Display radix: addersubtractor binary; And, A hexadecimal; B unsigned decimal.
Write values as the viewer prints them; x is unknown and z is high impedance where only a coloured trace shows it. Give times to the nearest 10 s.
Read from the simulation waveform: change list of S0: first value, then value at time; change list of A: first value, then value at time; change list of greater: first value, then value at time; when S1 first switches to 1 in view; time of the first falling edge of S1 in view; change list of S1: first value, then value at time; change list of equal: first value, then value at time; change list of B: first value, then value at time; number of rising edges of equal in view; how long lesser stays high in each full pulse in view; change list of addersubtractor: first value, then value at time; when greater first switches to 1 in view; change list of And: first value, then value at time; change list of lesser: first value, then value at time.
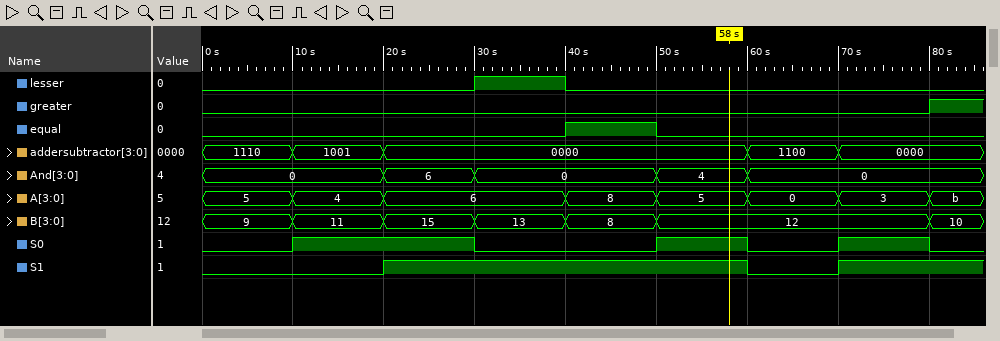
0, 1 at 10 s, 0 at 30 s, 1 at 50 s, 0 at 60 s, 1 at 70 s, 0 at 80 s
5, 4 at 10 s, 6 at 20 s, 8 at 40 s, 5 at 50 s, 0 at 60 s, 3 at 70 s, b at 80 s
0, 1 at 80 s
20 s
60 s
0, 1 at 20 s, 0 at 60 s, 1 at 70 s
0, 1 at 40 s, 0 at 50 s
9, 11 at 10 s, 15 at 20 s, 13 at 30 s, 8 at 40 s, 12 at 50 s, 10 at 80 s
1
10 s
1110, 1001 at 10 s, 0000 at 20 s, 1100 at 60 s, 0000 at 70 s
80 s
0, 6 at 20 s, 0 at 30 s, 4 at 50 s, 0 at 60 s
0, 1 at 30 s, 0 at 40 s
